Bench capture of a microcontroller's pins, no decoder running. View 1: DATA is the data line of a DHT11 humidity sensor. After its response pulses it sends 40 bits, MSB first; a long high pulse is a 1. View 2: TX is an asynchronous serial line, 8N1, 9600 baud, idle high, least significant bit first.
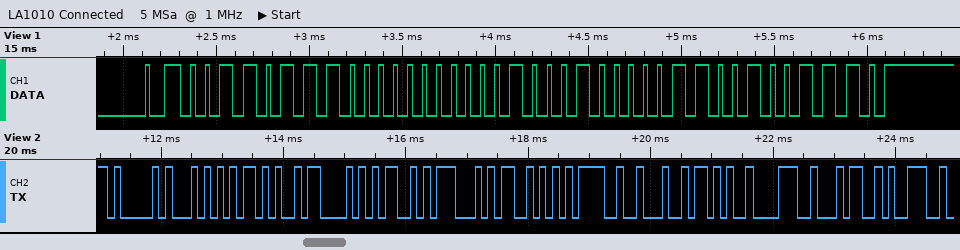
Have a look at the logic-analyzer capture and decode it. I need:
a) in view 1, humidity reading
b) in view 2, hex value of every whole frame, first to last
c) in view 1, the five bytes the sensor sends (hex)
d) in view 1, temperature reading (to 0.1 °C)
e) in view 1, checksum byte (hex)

55 %
41 54 2B 43 4D 47 53 3D 22 2B 38 34 39
37 00 11 06 4E
17.6 °C
0x4E
